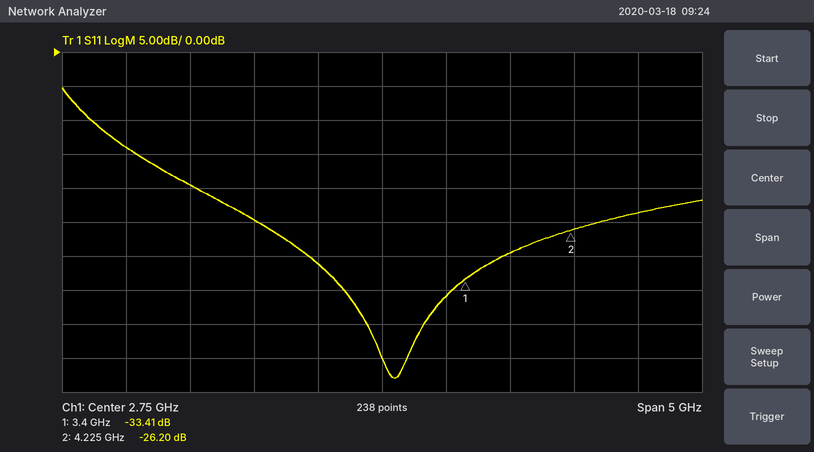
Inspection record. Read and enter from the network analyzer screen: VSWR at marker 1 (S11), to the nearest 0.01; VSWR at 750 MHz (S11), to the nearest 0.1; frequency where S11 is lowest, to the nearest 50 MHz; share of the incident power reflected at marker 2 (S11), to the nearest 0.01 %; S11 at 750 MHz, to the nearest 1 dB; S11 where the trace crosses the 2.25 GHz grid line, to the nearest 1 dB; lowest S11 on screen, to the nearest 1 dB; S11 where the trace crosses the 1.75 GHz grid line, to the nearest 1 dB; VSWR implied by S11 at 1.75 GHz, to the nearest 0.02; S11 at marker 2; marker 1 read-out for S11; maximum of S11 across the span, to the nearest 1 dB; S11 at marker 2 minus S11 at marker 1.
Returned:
1.04
1.5
2.85 GHz
0.24 %
-14 dB
-31 dB
-48 dB
-25 dB
1.12
-26.20 dB
-33.41 dB
-5 dB
7.21 dB
